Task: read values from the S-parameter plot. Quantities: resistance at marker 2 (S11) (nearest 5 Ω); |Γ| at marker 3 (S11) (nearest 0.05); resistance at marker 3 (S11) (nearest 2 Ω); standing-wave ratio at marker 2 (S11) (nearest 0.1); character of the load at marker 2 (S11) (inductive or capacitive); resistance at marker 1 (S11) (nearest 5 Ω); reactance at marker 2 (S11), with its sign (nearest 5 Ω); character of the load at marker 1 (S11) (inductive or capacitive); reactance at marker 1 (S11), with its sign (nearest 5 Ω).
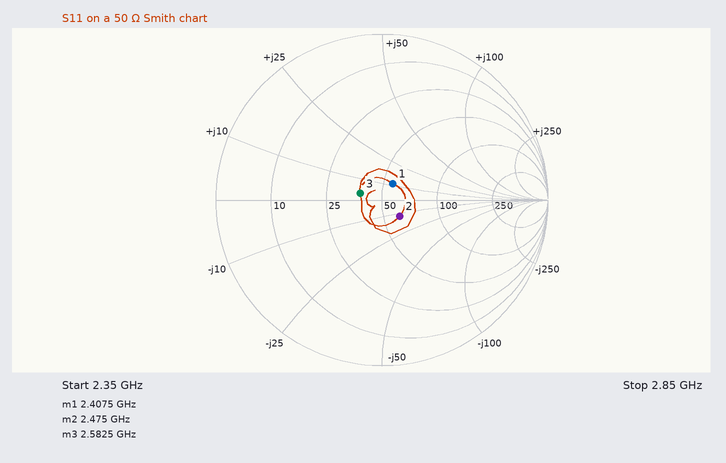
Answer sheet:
60 Ω
0.15
38 Ω
1.3
capacitive
55 Ω
-10 Ω
inductive
+10 Ω
